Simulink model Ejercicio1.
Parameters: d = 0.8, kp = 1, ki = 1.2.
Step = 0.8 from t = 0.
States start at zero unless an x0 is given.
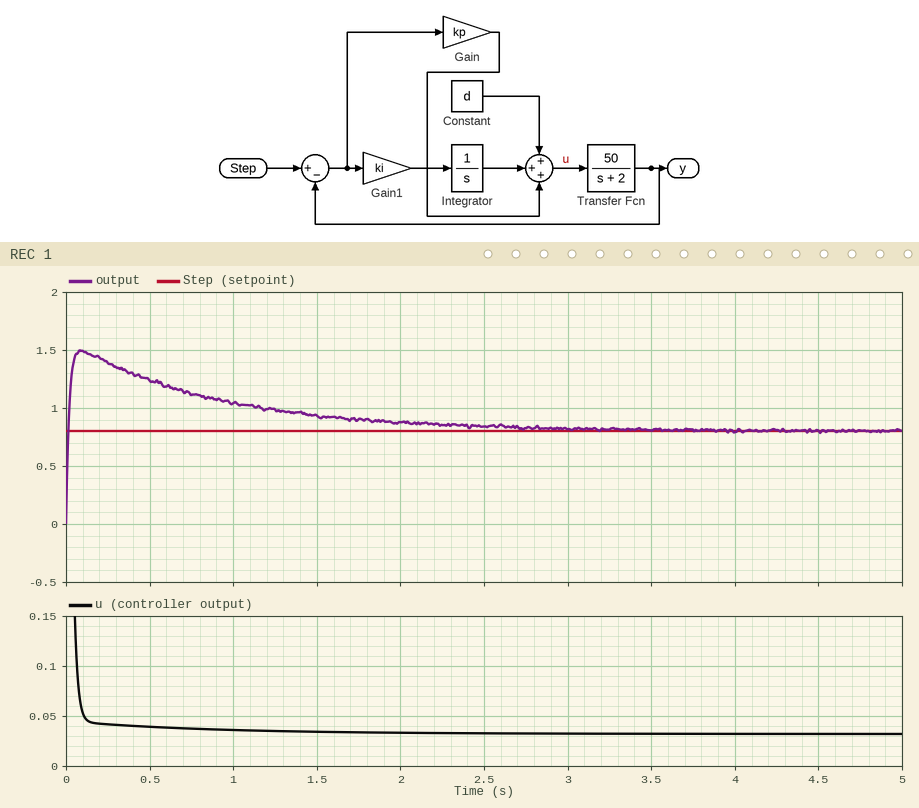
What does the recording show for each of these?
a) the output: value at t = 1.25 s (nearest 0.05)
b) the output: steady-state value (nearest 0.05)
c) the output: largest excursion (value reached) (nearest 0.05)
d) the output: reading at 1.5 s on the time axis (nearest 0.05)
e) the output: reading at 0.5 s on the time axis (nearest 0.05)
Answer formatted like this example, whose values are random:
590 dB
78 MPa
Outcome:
1.00
0.80
1.50
0.95
1.25
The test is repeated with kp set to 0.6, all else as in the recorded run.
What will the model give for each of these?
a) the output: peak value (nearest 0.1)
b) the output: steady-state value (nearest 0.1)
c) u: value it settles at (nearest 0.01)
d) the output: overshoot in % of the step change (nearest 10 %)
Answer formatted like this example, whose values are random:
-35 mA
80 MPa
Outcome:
1.9
0.8
0.03
130 %
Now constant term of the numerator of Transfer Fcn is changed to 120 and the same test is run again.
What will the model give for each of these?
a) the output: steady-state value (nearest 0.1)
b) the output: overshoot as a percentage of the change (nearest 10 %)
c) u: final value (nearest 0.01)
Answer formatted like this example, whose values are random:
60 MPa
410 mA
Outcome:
0.8
90 %
0.01
